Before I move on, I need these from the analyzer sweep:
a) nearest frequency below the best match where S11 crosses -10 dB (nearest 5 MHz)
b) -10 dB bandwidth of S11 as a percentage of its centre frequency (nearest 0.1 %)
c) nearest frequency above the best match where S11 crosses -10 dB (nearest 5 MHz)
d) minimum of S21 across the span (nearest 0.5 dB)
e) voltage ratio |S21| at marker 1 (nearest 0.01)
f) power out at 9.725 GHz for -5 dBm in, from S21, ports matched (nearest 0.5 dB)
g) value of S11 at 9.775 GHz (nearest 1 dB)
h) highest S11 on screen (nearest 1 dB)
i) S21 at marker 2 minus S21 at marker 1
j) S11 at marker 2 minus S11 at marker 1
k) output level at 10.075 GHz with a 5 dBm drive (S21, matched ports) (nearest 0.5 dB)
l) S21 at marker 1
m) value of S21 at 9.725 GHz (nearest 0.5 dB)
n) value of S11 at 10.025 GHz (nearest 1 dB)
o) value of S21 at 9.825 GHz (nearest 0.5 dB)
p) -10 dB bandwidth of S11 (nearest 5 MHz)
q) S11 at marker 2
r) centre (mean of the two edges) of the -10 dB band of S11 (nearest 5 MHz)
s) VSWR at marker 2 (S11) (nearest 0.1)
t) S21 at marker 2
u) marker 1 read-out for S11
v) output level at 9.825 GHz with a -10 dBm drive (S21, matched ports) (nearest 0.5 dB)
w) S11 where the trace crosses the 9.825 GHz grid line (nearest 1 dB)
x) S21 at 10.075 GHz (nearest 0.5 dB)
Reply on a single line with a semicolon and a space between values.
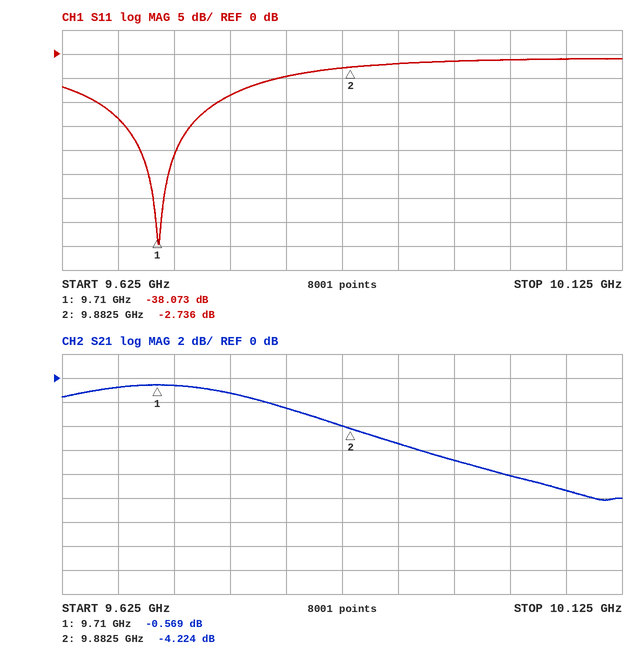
9.655 GHz; 1.1 %; 9.765 GHz; -10.0 dB; 0.94; -5.5 dBm; -9 dB; -1 dB; -3.655 dB; 35.337 dB; -4.5 dBm; -0.569 dB; -0.5 dB; -1 dB; -2.5 dB; 110 MHz; -2.736 dB; 9.710 GHz; 6.4; -4.224 dB; -38.073 dB; -12.5 dBm; -5 dB; -9.5 dB
